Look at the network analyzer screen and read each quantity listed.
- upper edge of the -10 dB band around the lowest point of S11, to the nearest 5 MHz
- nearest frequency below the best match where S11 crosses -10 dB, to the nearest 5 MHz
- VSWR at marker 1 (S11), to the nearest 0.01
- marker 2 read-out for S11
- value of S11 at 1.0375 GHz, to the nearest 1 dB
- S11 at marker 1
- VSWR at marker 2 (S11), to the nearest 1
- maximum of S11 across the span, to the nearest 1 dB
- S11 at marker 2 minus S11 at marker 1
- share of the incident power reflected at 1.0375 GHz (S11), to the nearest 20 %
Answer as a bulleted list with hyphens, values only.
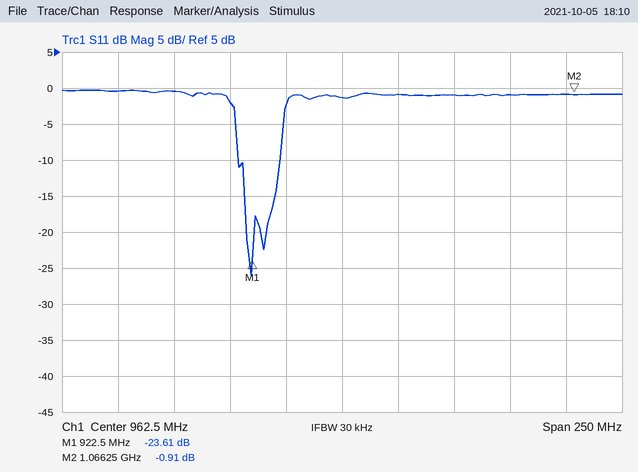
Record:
- 935 MHz
- 915 MHz
- 1.14
- -0.91 dB
- -1 dB
- -23.61 dB
- 19
- 0 dB
- 22.70 dB
- 80 %
